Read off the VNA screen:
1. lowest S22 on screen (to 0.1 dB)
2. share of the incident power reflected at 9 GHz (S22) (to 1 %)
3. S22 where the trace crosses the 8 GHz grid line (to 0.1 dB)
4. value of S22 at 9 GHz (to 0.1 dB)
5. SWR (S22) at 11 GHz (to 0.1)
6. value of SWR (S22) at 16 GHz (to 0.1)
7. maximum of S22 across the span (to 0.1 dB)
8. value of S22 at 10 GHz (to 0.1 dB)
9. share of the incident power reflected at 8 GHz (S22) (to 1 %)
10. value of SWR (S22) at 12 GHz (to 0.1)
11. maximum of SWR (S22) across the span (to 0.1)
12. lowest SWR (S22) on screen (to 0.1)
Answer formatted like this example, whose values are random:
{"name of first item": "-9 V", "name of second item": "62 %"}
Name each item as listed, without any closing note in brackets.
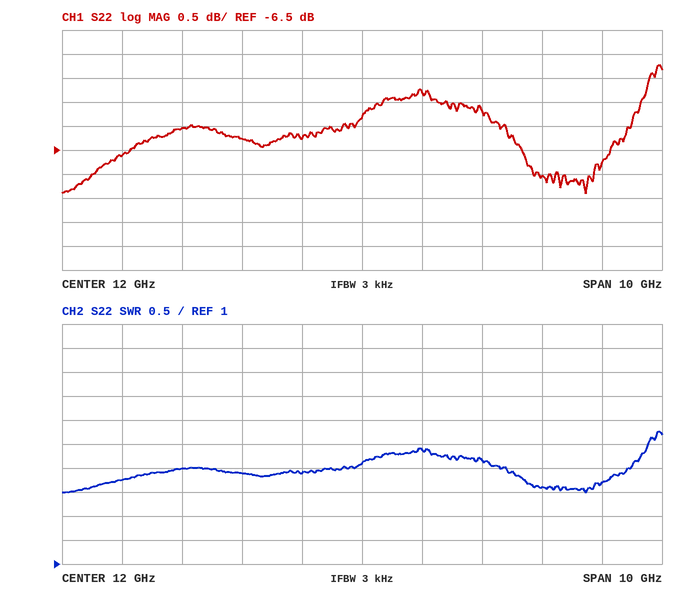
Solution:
{"lowest S22 on screen": "-7.4 dB", "share of the incident power reflected at 9 GHz (S22)": "25 %", "S22 where the trace crosses the 8 GHz grid line": "-6.6 dB", "value of S22 at 9 GHz": "-6.0 dB", "SWR (S22) at 11 GHz": "2.9", "value of SWR (S22) at 16 GHz": "2.7", "maximum of S22 across the span": "-4.7 dB", "value of S22 at 10 GHz": "-6.3 dB", "share of the incident power reflected at 8 GHz (S22)": "22 %", "value of SWR (S22) at 12 GHz": "3.1", "maximum of SWR (S22) across the span": "3.8", "lowest SWR (S22) on screen": "2.5"}
